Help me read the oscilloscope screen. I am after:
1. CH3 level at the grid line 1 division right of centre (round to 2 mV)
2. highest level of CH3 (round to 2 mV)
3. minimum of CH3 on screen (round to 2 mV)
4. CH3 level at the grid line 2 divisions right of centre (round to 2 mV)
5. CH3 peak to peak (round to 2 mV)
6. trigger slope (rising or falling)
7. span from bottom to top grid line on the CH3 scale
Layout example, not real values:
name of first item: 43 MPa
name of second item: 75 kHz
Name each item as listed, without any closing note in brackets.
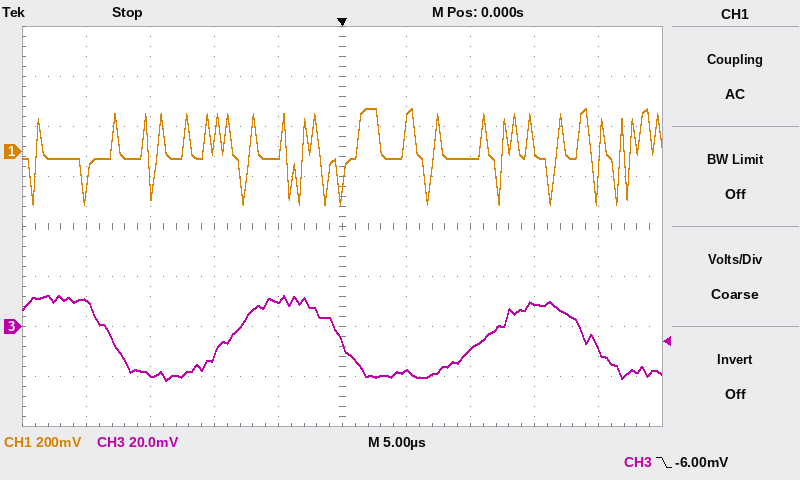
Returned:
CH3 level at the grid line 1 division right of centre: -18 mV
highest level of CH3: 12 mV
minimum of CH3 on screen: -22 mV
CH3 level at the grid line 2 divisions right of centre: -10 mV
CH3 peak to peak: 34 mV
trigger slope: falling
span from bottom to top grid line on the CH3 scale: 160 mV
